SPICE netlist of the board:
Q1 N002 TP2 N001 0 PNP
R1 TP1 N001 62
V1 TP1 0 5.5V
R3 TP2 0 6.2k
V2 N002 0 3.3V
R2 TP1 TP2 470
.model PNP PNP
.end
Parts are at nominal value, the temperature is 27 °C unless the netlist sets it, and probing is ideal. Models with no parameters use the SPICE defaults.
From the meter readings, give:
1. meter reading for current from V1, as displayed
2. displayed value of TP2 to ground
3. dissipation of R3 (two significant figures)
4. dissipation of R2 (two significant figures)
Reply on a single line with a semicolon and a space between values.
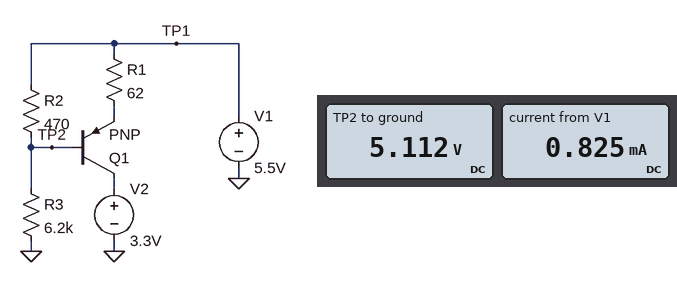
0.825 mA; 5.112 V; 4.2 mW; 320 µW
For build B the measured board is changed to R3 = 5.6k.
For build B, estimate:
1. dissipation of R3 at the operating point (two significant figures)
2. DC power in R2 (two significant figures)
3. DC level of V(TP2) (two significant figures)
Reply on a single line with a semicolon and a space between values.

4.6 mW; 390 µW; 5.1 V
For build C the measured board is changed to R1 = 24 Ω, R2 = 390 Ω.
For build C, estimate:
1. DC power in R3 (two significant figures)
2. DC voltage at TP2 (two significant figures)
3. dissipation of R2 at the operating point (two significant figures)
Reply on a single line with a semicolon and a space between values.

4.3 mW; 5.2 V; 270 µW
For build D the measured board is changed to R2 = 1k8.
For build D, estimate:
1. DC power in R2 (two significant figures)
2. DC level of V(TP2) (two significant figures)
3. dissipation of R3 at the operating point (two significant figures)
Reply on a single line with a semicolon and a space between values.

750 µW; 4.3 V; 3.0 mW
